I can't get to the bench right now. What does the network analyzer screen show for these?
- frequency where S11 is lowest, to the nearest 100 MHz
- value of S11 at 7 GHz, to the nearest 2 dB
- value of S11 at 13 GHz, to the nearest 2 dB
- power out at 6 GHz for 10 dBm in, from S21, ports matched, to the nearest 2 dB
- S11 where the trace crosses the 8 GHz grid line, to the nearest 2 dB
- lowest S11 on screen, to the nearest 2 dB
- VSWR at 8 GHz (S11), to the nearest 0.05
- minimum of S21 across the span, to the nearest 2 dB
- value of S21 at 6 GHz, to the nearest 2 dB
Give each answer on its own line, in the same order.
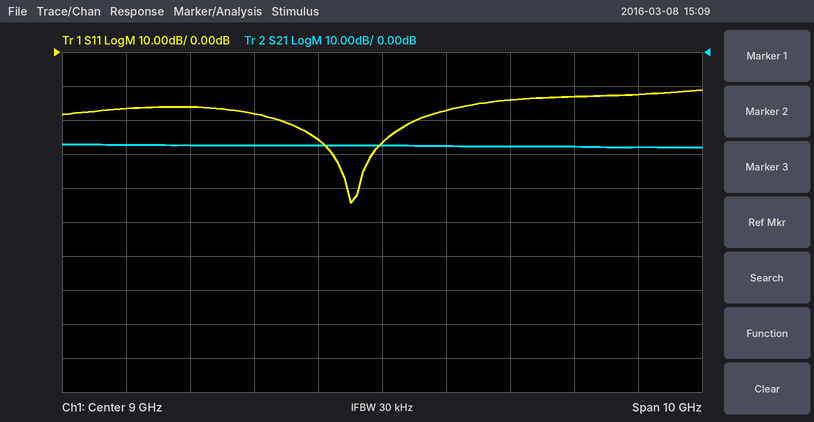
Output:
8.5 GHz
-18 dB
-12 dB
-18 dBm
-26 dB
-44 dB
1.10
-28 dB
-28 dB
